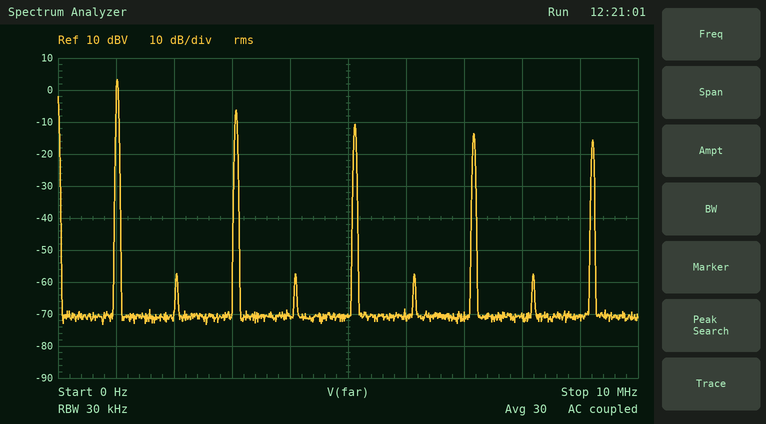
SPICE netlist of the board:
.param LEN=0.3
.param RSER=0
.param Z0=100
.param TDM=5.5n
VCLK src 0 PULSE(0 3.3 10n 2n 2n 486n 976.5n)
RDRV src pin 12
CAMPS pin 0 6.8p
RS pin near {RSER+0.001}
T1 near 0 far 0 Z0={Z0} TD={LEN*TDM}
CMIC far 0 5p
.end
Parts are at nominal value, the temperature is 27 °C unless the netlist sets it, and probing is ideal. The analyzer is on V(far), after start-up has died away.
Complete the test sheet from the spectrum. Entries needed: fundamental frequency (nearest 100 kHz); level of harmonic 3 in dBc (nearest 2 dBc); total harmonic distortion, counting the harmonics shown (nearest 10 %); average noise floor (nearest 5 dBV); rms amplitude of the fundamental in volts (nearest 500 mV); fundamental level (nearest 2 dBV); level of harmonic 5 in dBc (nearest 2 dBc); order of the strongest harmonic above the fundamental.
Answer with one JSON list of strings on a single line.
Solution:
["1.0 MHz", "-10 dBc", "40 %", "-70 dBV", "1.5 V", "4 dBV", "-14 dBc", "3"]
